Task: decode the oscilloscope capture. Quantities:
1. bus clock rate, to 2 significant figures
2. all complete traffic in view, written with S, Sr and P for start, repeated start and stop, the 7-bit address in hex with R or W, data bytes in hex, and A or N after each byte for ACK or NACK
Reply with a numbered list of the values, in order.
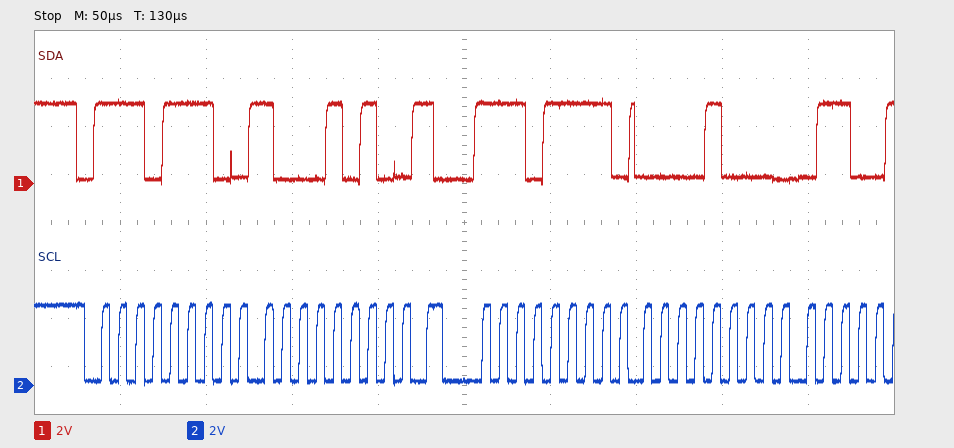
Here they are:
1. 100 kHz
2. S 77W A 8A A Sr 77R A 08 A
